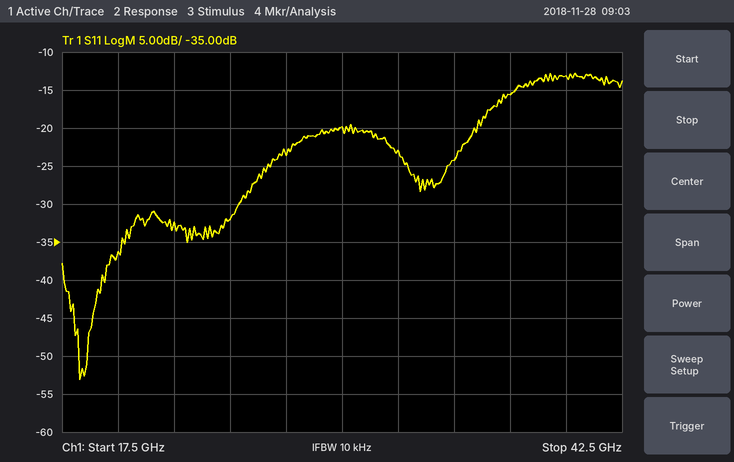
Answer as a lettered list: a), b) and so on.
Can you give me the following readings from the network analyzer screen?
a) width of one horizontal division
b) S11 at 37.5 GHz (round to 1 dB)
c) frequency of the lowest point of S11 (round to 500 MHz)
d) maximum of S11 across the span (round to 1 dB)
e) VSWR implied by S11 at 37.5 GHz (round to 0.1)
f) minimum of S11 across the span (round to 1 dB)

a) 2.5 GHz
b) -16 dB
c) 18.5 GHz
d) -13 dB
e) 1.4
f) -53 dB
